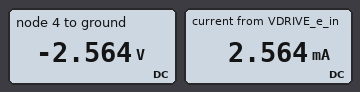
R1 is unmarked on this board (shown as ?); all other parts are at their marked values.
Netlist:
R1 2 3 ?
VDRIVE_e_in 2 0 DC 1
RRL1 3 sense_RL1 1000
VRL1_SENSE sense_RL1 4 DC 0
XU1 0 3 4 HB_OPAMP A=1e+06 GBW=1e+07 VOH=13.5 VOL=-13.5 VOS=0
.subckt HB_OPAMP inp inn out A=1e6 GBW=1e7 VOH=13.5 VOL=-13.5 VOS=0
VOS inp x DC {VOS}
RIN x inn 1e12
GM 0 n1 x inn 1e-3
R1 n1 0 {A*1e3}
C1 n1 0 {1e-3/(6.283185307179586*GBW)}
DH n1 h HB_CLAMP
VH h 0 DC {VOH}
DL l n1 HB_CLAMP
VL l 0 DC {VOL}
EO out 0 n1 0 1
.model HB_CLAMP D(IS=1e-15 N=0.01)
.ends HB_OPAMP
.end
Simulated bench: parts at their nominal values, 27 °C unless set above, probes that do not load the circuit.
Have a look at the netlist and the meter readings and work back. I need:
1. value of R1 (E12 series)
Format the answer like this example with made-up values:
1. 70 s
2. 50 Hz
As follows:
1. 390 Ω
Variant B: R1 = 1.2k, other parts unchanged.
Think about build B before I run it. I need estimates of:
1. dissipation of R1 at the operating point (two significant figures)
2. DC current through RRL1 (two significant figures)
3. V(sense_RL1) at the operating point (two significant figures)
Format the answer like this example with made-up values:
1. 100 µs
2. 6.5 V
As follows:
1. 830 µW
2. 830 µA
3. -830 mV
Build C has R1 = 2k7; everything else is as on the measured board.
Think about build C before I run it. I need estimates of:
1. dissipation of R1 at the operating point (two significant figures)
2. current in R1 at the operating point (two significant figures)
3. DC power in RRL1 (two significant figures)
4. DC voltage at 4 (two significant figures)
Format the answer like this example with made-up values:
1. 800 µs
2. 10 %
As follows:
1. 370 µW
2. 370 µA
3. 140 µW
4. -370 mV
